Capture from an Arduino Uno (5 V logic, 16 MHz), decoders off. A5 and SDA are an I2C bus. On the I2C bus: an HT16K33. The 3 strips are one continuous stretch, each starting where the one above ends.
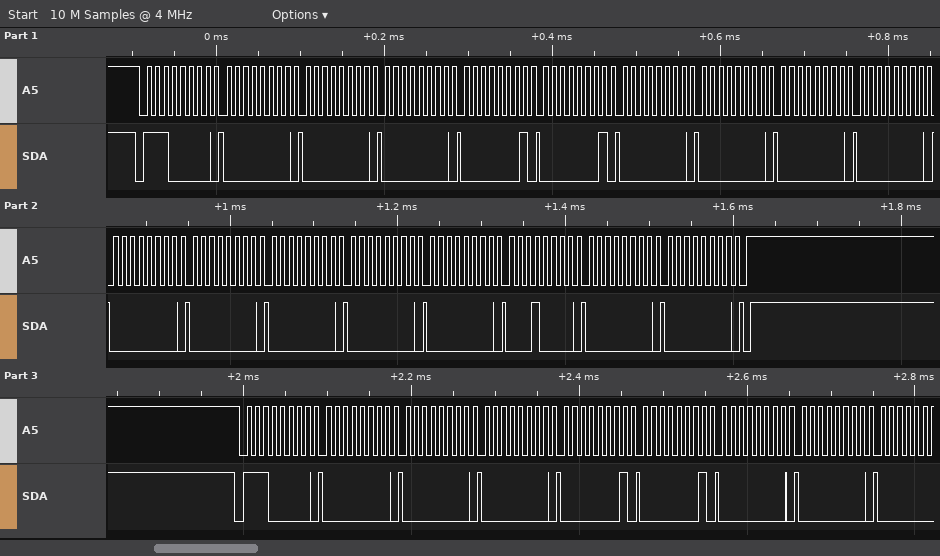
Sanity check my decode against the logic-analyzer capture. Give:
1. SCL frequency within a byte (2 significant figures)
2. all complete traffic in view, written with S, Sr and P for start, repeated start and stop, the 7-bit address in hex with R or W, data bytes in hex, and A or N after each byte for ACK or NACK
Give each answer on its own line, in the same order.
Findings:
100 kHz
S 70W A 00 A 00 A 00 A 01 A 01 A 00 A 00 A 00 A 00 A 00 A 00 A 00 A 00 A 00 A 10 A 00 A 00 A P S 70W A 00 A 00 A 00 A 01 A 01 A 00 A 00 A
